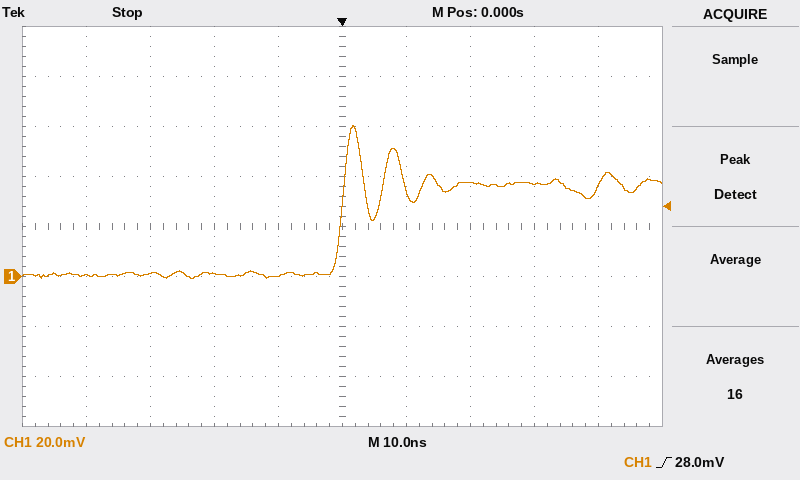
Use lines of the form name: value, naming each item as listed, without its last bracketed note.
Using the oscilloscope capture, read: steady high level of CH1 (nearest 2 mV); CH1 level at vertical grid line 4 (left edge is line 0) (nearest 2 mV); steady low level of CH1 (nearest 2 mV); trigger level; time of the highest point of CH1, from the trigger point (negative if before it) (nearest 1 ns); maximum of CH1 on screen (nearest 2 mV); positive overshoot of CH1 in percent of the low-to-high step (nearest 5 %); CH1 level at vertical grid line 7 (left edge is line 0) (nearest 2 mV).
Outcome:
steady high level of CH1: 38 mV
CH1 level at vertical grid line 4 (left edge is line 0): 0 mV
steady low level of CH1: 0 mV
trigger level: 28.0 mV
time of the highest point of CH1, from the trigger point (negative if before it): +2 ns
maximum of CH1 on screen: 60 mV
positive overshoot of CH1 in percent of the low-to-high step: 65 %
CH1 level at vertical grid line 7 (left edge is line 0): 38 mV
